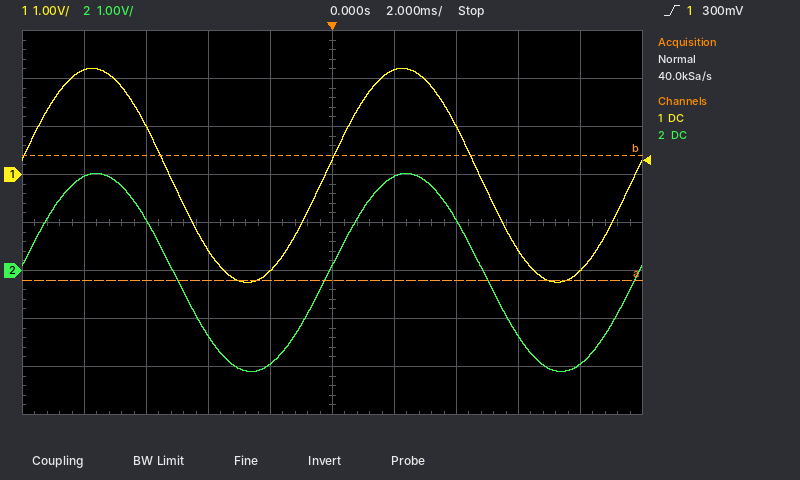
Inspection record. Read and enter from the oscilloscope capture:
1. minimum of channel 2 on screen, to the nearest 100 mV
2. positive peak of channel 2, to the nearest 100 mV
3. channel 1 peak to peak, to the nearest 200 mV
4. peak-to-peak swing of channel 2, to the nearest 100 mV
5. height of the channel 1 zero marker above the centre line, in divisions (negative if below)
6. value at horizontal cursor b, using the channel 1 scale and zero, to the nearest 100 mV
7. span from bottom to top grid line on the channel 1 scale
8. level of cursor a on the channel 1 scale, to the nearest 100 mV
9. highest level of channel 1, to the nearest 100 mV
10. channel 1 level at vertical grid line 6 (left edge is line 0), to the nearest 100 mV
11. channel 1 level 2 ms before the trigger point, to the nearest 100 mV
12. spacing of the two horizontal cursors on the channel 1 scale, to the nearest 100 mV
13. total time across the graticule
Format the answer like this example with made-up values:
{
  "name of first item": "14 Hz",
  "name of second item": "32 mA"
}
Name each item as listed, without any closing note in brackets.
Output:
{
  "minimum of channel 2 on screen, to the nearest 100 mV": "-2.1 V",
  "positive peak of channel 2, to the nearest 100 mV": "2.0 V",
  "channel 1 peak to peak, to the nearest 200 mV": "4.4 V",
  "peak-to-peak swing of channel 2, to the nearest 100 mV": "4.1 V",
  "height of the channel 1 zero marker above the centre line, in divisions": "+1.0 div",
  "value at horizontal cursor b, using the channel 1 scale and zero, to the nearest 100 mV": "400 mV",
  "span from bottom to top grid line on the channel 1 scale": "8 V",
  "level of cursor a on the channel 1 scale, to the nearest 100 mV": "-2.2 V",
  "highest level of channel 1, to the nearest 100 mV": "2.2 V",
  "channel 1 level at vertical grid line 6 (left edge is line 0), to the nearest 100 mV": "2.2 V",
  "channel 1 level 2 ms before the trigger point, to the nearest 100 mV": "-2.0 V",
  "spacing of the two horizontal cursors on the channel 1 scale, to the nearest 100 mV": "2.6 V",
  "total time across the graticule": "20 ms"
}
